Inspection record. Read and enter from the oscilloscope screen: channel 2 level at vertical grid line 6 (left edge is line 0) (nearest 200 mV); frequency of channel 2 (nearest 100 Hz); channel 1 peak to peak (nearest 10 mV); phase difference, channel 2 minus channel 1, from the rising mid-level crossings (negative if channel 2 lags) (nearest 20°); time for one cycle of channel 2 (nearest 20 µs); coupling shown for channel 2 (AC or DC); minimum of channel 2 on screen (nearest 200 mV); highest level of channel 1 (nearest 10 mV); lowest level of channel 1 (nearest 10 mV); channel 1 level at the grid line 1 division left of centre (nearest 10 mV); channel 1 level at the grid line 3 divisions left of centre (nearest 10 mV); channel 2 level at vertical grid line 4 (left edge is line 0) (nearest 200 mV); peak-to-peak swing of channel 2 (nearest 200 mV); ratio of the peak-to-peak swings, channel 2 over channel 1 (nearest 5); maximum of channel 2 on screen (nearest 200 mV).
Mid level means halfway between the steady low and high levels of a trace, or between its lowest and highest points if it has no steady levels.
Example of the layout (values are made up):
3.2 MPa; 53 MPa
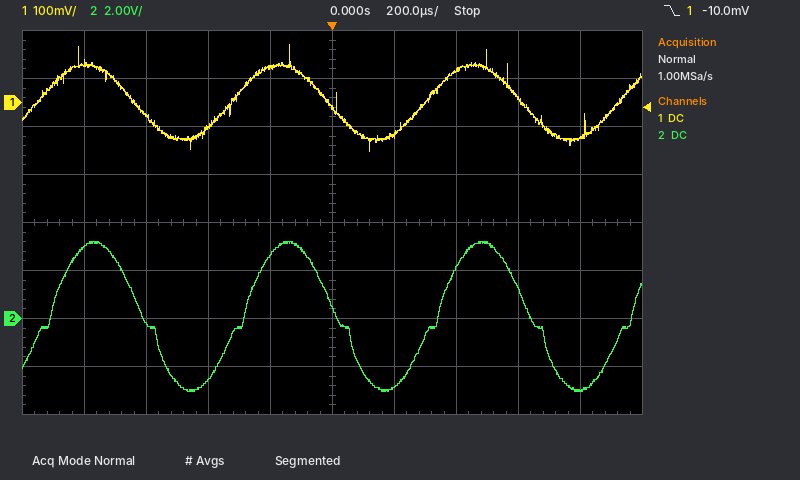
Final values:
-2.8 V; 1.6 kHz; 220 mV; -20°; 620 µs; DC; -3.0 V; 120 mV; -100 mV; 70 mV; -30 mV; 2.6 V; 6.2 V; 30; 3.2 V
